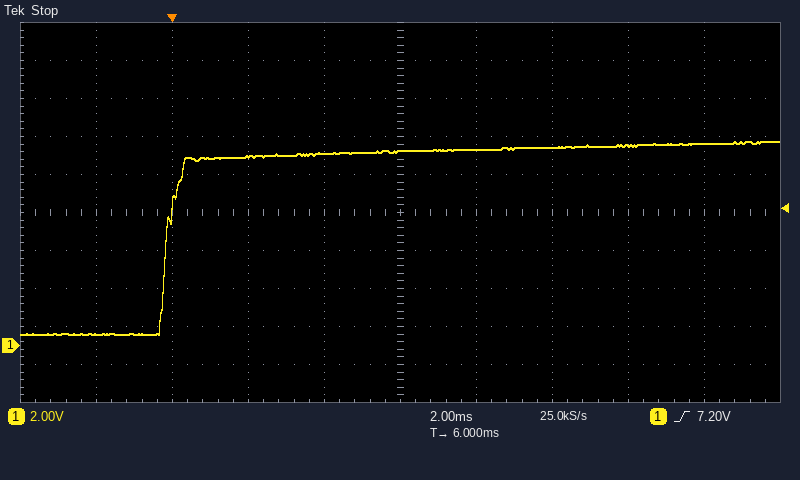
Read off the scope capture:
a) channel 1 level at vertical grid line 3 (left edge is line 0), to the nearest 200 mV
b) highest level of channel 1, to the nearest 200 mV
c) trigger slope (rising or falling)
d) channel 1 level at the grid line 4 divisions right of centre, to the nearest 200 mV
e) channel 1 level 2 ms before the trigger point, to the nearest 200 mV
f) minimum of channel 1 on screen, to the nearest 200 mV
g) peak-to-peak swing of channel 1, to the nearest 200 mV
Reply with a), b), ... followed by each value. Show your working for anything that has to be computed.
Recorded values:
a) 10.0 V
b) 10.8 V
c) rising
d) 10.6 V
e) 600 mV
f) 600 mV
g) 10.8 V − (600 mV) = 10.2 V
